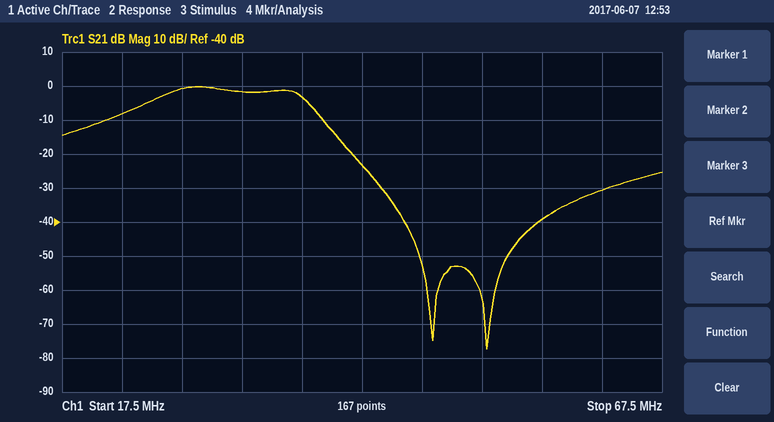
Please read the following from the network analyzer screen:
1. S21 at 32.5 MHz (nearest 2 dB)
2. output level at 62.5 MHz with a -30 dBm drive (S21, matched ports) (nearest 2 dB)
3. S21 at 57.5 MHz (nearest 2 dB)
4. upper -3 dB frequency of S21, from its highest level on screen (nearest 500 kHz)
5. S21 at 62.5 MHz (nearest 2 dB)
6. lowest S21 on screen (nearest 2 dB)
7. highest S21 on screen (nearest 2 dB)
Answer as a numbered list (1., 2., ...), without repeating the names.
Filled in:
1. -2 dB
2. -60 dBm
3. -40 dB
4. 37.5 MHz
5. -30 dB
6. -78 dB
7. 0 dB
